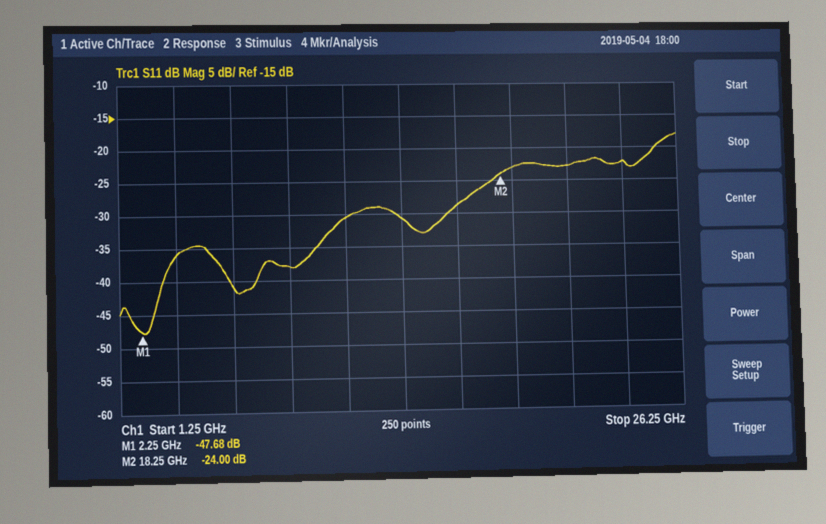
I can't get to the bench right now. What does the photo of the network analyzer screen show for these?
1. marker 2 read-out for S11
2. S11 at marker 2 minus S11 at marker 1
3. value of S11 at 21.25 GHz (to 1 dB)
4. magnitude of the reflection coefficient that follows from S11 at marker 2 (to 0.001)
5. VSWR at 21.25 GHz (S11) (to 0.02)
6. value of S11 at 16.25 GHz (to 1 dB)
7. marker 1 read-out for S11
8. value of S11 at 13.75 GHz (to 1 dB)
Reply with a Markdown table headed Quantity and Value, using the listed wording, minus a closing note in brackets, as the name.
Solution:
| Quantity | Value |
|---|---|
| marker 2 read-out for S11 | -24.00 dB |
| S11 at marker 2 minus S11 at marker 1 | 23.68 dB |
| value of S11 at 21.25 GHz | -23 dB |
| magnitude of the reflection coefficient that follows from S11 at marker 2 | 0.063 |
| VSWR at 21.25 GHz (S11) | 1.16 |
| value of S11 at 16.25 GHz | -29 dB |
| marker 1 read-out for S11 | -47.68 dB |
| value of S11 at 13.75 GHz | -31 dB |
